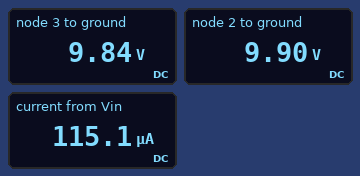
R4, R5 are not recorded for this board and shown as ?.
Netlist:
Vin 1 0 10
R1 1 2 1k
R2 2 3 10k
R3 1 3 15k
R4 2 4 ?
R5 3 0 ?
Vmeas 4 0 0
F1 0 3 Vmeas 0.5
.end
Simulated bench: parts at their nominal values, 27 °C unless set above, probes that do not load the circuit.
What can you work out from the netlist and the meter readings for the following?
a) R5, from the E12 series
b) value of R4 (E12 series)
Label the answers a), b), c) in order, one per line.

a) 150 kΩ
b) 100 kΩ
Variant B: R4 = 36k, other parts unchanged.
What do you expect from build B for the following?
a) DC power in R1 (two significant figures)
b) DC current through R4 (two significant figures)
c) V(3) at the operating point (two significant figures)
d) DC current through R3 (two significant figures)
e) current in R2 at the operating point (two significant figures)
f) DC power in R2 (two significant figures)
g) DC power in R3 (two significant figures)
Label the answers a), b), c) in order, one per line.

a) 49 µW
b) 270 µA
c) 10 V
d) 18 µA
e) 49 µA
f) 24 µW
g) 4.9 µW
